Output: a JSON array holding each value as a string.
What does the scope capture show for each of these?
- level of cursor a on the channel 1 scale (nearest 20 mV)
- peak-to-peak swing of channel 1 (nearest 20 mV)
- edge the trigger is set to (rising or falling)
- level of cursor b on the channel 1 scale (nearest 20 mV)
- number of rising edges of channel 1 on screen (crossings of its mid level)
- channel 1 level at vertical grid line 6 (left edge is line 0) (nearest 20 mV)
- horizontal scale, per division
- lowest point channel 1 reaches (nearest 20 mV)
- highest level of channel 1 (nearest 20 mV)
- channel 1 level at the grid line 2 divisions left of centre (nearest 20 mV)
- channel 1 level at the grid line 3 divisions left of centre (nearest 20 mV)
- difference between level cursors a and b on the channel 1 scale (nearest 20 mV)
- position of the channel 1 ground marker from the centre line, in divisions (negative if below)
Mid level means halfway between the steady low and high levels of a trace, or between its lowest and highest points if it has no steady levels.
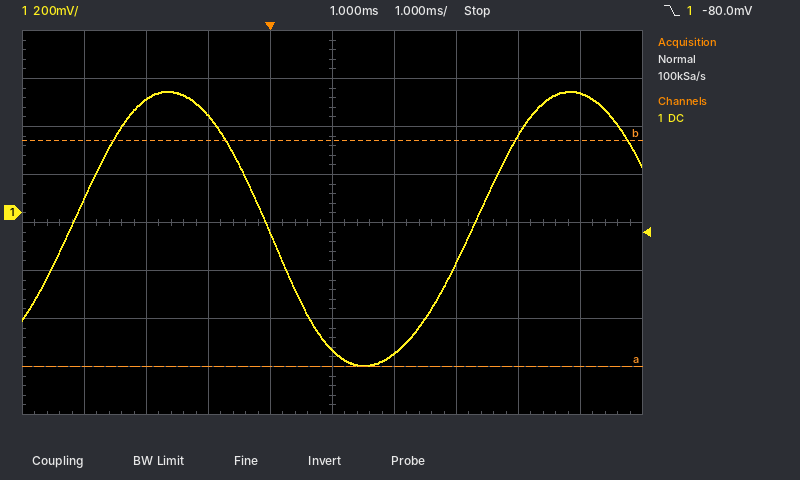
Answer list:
["-640 mV", "1.14 V", "falling", "300 mV", "2", "-580 mV", "1 ms", "-640 mV", "500 mV", "400 mV", "480 mV", "940 mV", "+0.2 div"]
